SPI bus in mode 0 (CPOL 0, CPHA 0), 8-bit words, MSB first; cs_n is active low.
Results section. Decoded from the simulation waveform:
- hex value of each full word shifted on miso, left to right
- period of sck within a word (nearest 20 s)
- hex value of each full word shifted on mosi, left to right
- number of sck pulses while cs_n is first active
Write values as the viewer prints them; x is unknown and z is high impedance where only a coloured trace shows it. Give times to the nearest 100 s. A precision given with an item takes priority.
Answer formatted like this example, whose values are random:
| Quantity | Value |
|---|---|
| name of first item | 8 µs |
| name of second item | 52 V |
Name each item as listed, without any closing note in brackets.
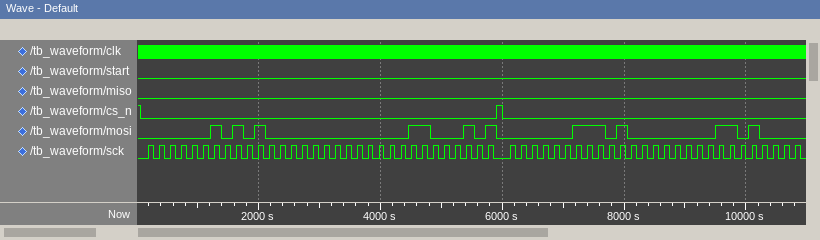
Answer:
| Quantity | Value |
|---|---|
| hex value of each full word shifted on miso, left to right | 00, 00, 00, 00, 00, 00, 00 |
| period of sck within a word | 180 s |
| hex value of each full word shifted on mosi, left to right | 02, A0, 00, C5, 03, A0, 1A |
| number of sck pulses while cs_n is first active | 32 |
